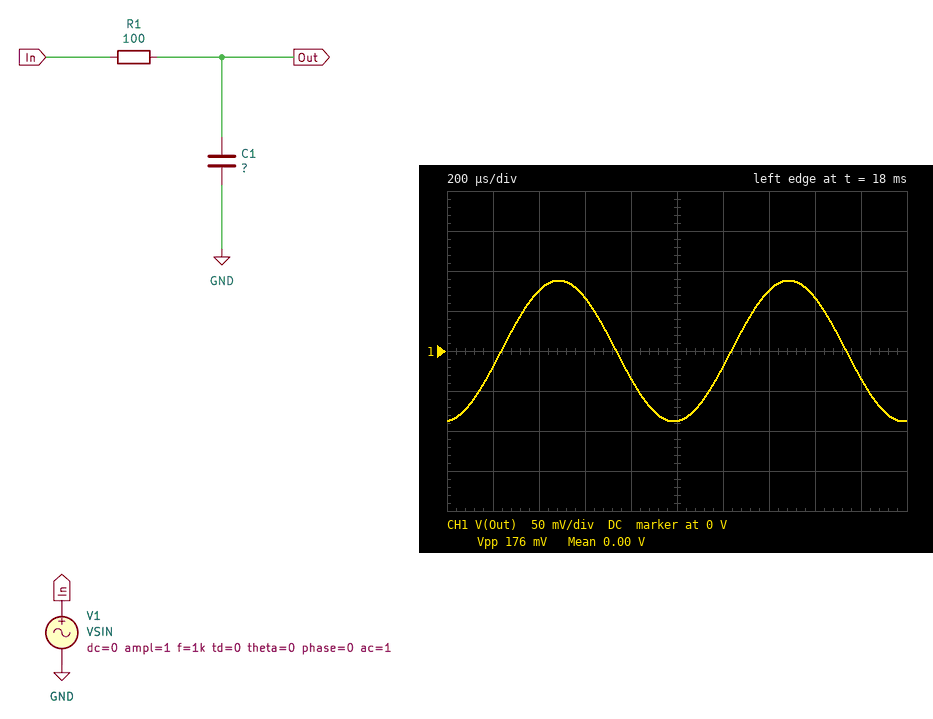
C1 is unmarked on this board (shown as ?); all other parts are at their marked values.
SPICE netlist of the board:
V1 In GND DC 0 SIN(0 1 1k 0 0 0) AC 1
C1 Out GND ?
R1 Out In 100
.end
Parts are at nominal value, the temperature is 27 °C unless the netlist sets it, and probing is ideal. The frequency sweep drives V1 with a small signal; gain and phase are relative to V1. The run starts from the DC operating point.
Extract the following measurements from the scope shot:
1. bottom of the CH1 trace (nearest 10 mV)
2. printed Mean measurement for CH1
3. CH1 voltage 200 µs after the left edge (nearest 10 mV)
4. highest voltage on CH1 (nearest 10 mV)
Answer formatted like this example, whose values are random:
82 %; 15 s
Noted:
-90 mV; 0.00 V; -20 mV; 90 mV
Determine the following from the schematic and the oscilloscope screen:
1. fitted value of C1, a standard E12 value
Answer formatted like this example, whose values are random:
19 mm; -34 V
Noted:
18 µF
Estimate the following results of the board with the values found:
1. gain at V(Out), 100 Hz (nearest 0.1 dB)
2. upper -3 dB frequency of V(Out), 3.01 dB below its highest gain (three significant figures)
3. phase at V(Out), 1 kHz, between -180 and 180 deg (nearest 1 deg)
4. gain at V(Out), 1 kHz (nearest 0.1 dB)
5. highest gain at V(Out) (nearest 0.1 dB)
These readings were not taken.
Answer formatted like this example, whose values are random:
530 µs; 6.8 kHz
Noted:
-3.6 dB; 88.4 Hz; -85 deg; -21.1 dB; 0 dB
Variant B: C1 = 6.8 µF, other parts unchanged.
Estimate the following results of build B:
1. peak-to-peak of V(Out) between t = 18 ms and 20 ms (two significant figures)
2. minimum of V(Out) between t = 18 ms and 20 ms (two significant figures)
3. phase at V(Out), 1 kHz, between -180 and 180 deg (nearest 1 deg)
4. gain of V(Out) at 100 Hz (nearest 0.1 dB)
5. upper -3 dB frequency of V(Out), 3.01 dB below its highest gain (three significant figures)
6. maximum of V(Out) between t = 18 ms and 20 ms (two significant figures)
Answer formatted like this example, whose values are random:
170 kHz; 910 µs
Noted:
460 mV; -230 mV; -77 deg; -0.7 dB; 234 Hz; 230 mV
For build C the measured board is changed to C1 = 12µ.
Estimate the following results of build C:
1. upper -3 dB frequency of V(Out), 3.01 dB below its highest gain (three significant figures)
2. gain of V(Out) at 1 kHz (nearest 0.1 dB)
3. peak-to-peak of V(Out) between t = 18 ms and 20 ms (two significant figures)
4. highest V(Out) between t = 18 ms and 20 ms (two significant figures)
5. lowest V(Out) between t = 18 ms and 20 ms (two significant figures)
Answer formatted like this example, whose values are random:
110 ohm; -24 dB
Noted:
133 Hz; -17.6 dB; 260 mV; 130 mV; -130 mV
